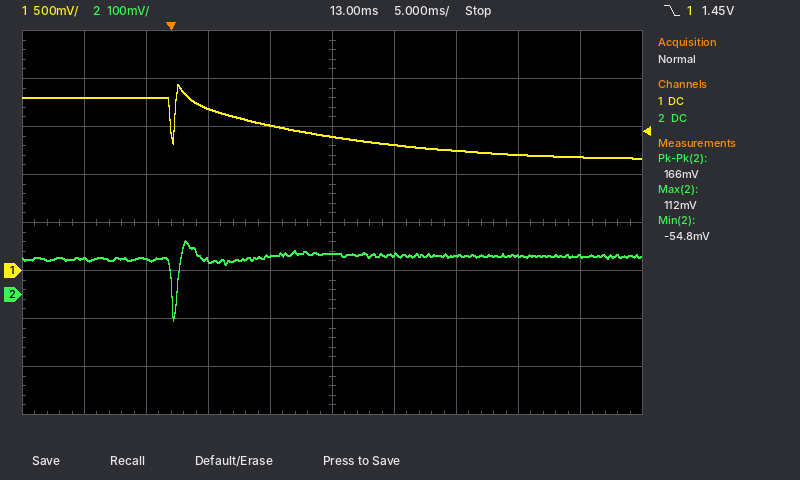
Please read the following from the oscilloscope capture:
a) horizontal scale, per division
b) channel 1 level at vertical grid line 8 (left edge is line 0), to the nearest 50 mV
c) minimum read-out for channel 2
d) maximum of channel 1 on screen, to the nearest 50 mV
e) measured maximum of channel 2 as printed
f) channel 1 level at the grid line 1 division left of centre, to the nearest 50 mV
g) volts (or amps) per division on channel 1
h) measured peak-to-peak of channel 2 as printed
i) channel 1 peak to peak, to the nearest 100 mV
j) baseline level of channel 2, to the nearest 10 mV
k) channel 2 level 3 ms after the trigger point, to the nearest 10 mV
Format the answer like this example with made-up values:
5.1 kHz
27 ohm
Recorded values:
5 ms
1.20 V
-54.8 mV
1.95 V
112 mV
1.50 V
500 mV
166 mV
800 mV
80 mV
70 mV
